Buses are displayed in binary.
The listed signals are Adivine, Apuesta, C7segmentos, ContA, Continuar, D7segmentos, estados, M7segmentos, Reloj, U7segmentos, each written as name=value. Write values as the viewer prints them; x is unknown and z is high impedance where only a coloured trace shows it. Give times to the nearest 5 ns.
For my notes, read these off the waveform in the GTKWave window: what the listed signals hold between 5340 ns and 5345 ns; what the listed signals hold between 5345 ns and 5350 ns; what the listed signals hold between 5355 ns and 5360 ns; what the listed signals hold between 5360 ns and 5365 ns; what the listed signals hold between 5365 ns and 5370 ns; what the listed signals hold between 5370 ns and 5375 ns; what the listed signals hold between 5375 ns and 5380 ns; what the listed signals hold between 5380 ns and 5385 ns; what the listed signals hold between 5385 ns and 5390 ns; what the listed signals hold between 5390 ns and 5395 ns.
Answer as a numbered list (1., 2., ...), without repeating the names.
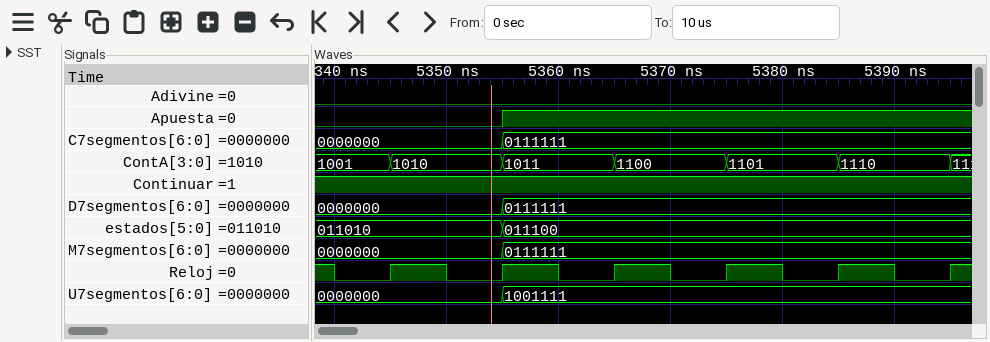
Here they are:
1. Adivine=0, Apuesta=0, C7segmentos=0000000, ContA=1001, Continuar=1, D7segmentos=0000000, estados=011010, M7segmentos=0000000, Reloj=0, U7segmentos=0000000
2. Adivine=0, Apuesta=0, C7segmentos=0000000, ContA=1010, Continuar=1, D7segmentos=0000000, estados=011010, M7segmentos=0000000, Reloj=1, U7segmentos=0000000
3. Adivine=0, Apuesta=1, C7segmentos=0111111, ContA=1011, Continuar=1, D7segmentos=0111111, estados=011100, M7segmentos=0111111, Reloj=1, U7segmentos=1001111
4. Adivine=0, Apuesta=1, C7segmentos=0111111, ContA=1011, Continuar=1, D7segmentos=0111111, estados=011100, M7segmentos=0111111, Reloj=0, U7segmentos=1001111
5. Adivine=0, Apuesta=1, C7segmentos=0111111, ContA=1100, Continuar=1, D7segmentos=0111111, estados=011100, M7segmentos=0111111, Reloj=1, U7segmentos=1001111
6. Adivine=0, Apuesta=1, C7segmentos=0111111, ContA=1100, Continuar=1, D7segmentos=0111111, estados=011100, M7segmentos=0111111, Reloj=0, U7segmentos=1001111
7. Adivine=0, Apuesta=1, C7segmentos=0111111, ContA=1101, Continuar=1, D7segmentos=0111111, estados=011100, M7segmentos=0111111, Reloj=1, U7segmentos=1001111
8. Adivine=0, Apuesta=1, C7segmentos=0111111, ContA=1101, Continuar=1, D7segmentos=0111111, estados=011100, M7segmentos=0111111, Reloj=0, U7segmentos=1001111
9. Adivine=0, Apuesta=1, C7segmentos=0111111, ContA=1110, Continuar=1, D7segmentos=0111111, estados=011100, M7segmentos=0111111, Reloj=1, U7segmentos=1001111
10. Adivine=0, Apuesta=1, C7segmentos=0111111, ContA=1110, Continuar=1, D7segmentos=0111111, estados=011100, M7segmentos=0111111, Reloj=0, U7segmentos=1001111
